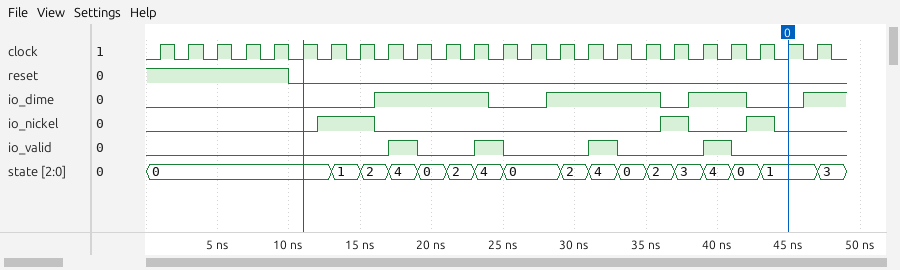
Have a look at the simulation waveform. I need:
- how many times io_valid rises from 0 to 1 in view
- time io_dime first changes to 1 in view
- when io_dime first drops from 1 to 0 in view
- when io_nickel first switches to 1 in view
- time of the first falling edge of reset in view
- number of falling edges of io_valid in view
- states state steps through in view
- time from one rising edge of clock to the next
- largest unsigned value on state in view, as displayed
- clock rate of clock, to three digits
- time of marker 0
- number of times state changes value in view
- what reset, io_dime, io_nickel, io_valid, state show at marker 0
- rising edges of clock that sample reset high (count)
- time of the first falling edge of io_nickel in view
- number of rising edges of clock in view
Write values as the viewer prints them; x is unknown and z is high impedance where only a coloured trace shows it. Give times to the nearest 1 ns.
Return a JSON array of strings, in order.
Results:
["4", "16 ns", "24 ns", "12 ns", "10 ns", "4", "0, 1, 2, 4, 0, 2, 4, 0, 2, 4, 0, 2, 3, 4, 0, 1, 3", "2 ns", "4", "500 MHz", "45 ns", "16", "reset=0, io_dime=0, io_nickel=0, io_valid=0, state=1", "5", "16 ns", "24"]
